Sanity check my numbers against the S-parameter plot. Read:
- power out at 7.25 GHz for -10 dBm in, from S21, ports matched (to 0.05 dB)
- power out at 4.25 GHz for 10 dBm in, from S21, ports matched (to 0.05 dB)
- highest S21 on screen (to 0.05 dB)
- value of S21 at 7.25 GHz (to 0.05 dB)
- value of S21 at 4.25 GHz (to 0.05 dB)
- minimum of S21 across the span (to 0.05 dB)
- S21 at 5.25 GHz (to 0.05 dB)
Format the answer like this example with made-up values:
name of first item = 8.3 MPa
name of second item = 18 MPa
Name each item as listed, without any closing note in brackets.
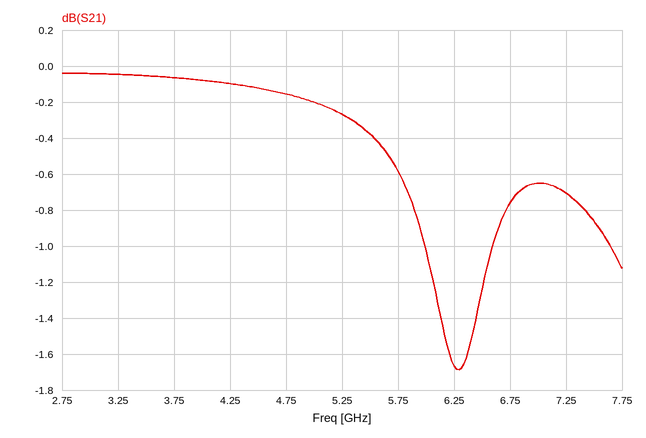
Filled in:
power out at 7.25 GHz for -10 dBm in, from S21, ports matched = -10.70 dBm
power out at 4.25 GHz for 10 dBm in, from S21, ports matched = 9.90 dBm
highest S21 on screen = -0.05 dB
value of S21 at 7.25 GHz = -0.70 dB
value of S21 at 4.25 GHz = -0.10 dB
minimum of S21 across the span = -1.70 dB
S21 at 5.25 GHz = -0.25 dB
